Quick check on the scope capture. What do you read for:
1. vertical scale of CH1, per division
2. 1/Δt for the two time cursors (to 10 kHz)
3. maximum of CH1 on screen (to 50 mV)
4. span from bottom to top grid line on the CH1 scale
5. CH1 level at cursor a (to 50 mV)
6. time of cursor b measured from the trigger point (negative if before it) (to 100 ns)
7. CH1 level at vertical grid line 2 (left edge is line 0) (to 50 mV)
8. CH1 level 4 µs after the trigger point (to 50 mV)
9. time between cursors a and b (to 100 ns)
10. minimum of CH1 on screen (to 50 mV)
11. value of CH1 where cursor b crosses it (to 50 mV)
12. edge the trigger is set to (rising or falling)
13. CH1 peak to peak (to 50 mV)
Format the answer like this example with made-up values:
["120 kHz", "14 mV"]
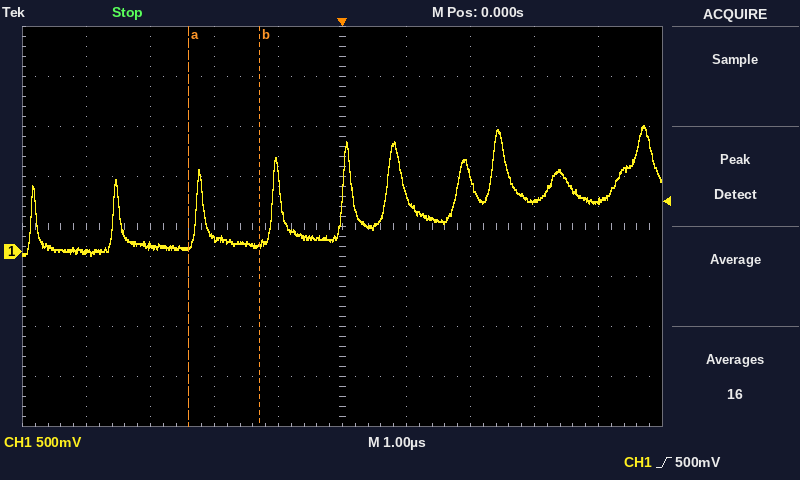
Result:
["500 mV", "910 kHz", "1.25 V", "4 V", "50 mV", "-1.3 µs", "50 mV", "500 mV", "1.1 µs", "-50 mV", "100 mV", "rising", "1.30 V"]
